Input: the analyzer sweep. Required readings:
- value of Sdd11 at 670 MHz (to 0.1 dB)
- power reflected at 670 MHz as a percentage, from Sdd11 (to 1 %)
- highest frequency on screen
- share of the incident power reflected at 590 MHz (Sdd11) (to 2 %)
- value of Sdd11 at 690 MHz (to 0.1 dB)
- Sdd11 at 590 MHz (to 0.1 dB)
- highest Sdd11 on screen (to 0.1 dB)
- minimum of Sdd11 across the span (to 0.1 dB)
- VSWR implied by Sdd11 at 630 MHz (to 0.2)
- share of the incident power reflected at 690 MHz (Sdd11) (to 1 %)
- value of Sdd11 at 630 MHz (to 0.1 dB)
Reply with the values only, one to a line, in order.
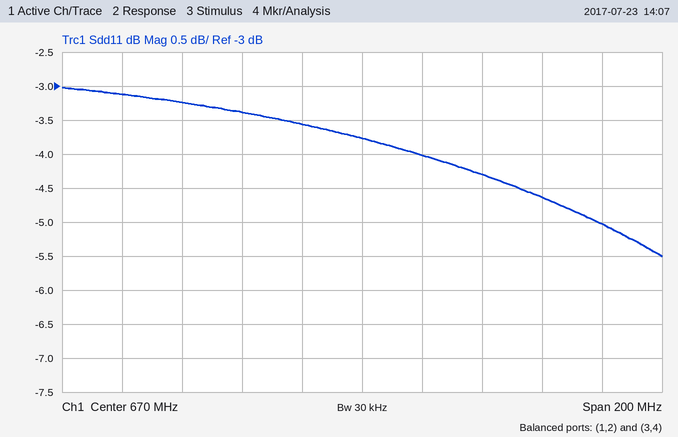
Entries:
-3.8 dB
42 %
770 MHz
48 %
-4.0 dB
-3.1 dB
-3.0 dB
-5.5 dB
5.2
40 %
-3.4 dB
